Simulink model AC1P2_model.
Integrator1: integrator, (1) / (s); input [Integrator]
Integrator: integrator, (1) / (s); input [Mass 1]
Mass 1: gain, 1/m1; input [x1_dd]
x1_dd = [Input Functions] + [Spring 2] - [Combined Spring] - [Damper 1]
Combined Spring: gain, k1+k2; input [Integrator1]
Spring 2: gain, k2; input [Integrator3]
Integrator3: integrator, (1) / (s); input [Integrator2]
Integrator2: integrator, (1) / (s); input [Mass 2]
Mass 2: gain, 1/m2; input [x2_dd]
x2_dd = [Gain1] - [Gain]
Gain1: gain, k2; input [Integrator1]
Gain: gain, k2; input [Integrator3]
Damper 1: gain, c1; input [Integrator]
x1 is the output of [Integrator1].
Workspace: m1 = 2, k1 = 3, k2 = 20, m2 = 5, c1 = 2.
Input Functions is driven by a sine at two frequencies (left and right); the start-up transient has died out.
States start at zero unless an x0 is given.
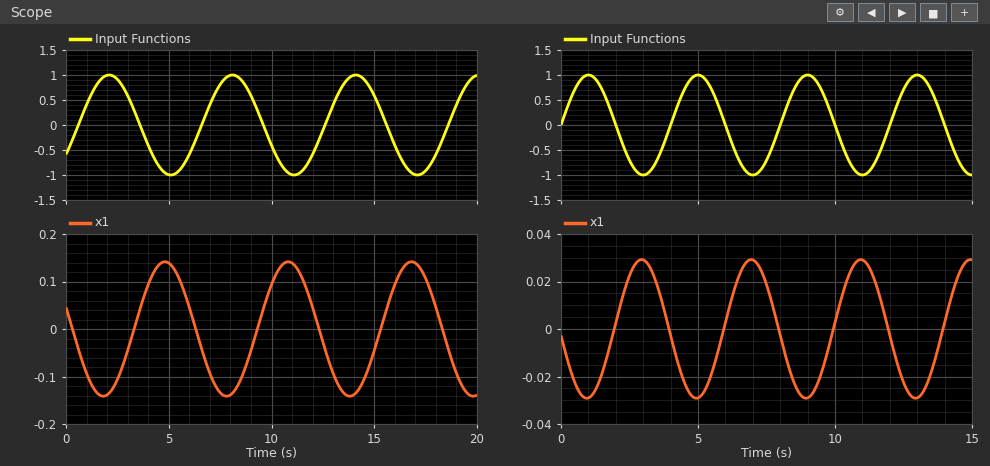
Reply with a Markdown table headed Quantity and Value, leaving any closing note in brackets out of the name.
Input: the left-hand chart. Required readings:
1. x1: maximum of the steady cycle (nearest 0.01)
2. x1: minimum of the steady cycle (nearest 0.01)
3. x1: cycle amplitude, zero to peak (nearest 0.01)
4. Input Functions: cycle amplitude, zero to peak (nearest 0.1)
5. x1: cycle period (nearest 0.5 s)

| Quantity | Value |
|---|---|
| x1: maximum of the steady cycle | 0.14 |
| x1: minimum of the steady cycle | -0.14 |
| x1: cycle amplitude, zero to peak | 0.14 |
| Input Functions: cycle amplitude, zero to peak | 1.0 |
| x1: cycle period | 6.0 s |
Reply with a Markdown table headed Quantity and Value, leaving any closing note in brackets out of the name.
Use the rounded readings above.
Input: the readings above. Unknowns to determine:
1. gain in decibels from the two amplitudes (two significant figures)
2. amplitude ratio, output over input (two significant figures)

| Quantity | Value |
|---|---|
| gain in decibels from the two amplitudes | -17 dB |
| amplitude ratio, output over input | 0.14 |
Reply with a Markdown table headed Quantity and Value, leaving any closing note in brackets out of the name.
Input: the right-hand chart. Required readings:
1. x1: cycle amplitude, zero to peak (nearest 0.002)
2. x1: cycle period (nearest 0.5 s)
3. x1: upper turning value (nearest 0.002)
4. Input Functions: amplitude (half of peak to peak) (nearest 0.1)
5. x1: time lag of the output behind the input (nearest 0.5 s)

| Quantity | Value |
|---|---|
| x1: cycle amplitude, zero to peak | 0.030 |
| x1: cycle period | 4.0 s |
| x1: upper turning value | 0.030 |
| Input Functions: amplitude (half of peak to peak) | 1.0 |
| x1: time lag of the output behind the input | 2.0 s |
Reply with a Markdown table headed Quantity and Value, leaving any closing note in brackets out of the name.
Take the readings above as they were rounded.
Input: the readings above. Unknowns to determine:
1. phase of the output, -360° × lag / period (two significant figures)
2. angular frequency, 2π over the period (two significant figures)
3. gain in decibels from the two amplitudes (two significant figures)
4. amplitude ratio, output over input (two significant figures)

| Quantity | Value |
|---|---|
| phase of the output, -360° × lag / period | -180° |
| angular frequency, 2π over the period | 1.6 rad/s |
| gain in decibels from the two amplitudes | -30 dB |
| amplitude ratio, output over input | 0.030 |
